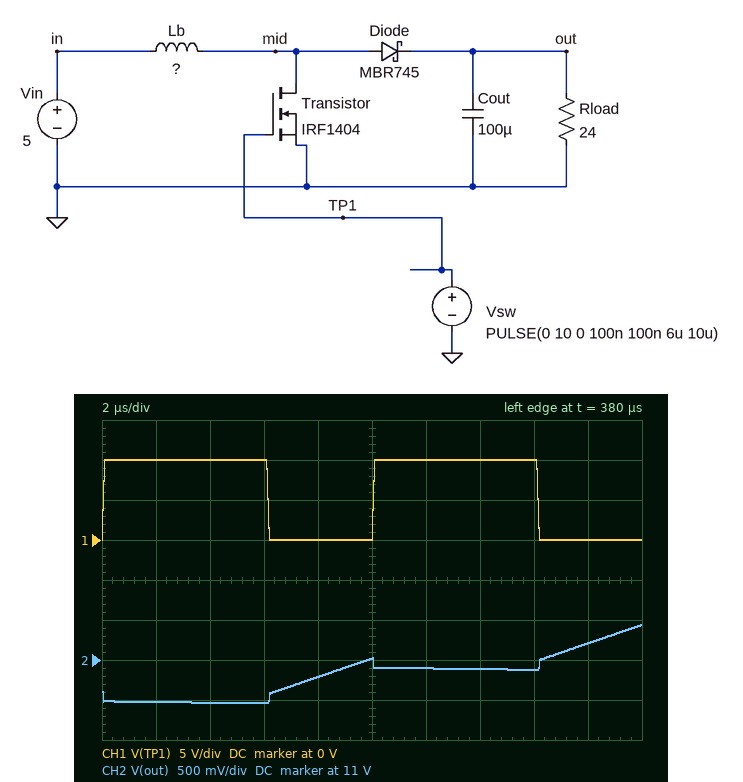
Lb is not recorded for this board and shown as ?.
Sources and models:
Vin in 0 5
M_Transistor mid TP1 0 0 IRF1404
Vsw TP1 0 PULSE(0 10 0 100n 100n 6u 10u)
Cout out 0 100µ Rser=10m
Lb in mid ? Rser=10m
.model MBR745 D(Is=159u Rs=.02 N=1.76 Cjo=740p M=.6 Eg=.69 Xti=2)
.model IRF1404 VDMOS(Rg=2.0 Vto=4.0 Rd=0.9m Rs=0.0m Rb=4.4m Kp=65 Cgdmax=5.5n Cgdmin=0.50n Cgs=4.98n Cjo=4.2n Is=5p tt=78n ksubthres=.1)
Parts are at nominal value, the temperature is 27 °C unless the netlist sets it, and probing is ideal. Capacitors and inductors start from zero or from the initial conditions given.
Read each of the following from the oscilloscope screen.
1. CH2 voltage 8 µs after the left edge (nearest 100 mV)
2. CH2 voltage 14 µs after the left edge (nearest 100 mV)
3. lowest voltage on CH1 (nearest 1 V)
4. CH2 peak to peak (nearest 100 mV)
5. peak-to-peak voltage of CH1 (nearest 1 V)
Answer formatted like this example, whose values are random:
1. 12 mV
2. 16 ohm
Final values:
1. 10.8 V
2. 10.9 V
3. 0 V
4. 1.0 V
5. 10 V
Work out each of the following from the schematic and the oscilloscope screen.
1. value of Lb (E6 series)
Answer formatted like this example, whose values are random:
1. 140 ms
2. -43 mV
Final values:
1. 100 µH
